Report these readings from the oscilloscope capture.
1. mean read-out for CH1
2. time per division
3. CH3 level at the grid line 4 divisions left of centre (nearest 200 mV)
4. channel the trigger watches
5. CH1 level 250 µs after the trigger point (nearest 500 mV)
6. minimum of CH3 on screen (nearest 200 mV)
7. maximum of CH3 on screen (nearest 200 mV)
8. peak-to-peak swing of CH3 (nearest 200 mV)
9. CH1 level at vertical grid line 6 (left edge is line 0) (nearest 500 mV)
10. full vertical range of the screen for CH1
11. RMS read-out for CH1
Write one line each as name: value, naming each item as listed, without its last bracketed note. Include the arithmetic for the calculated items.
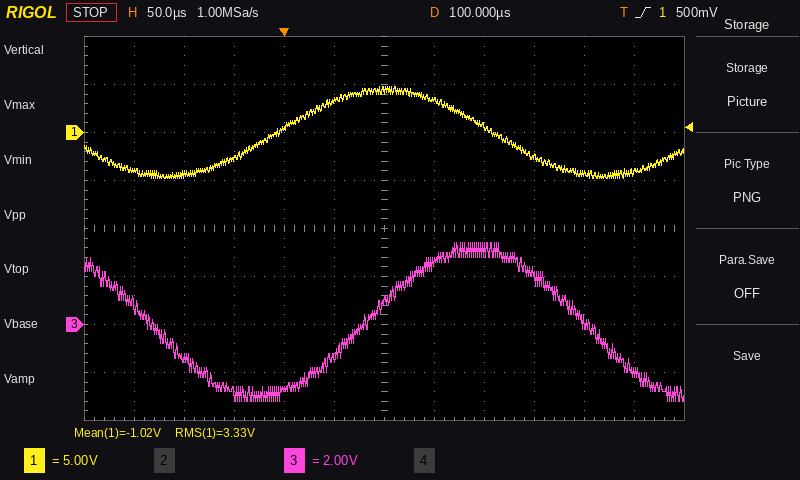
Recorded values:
mean read-out for CH1: -1.02 V
time per division: 50 µs
CH3 level at the grid line 4 divisions left of centre: -1.4 V
channel the trigger watches: CH1
CH1 level 250 µs after the trigger point: -2.5 V
minimum of CH3 on screen: -3.2 V
maximum of CH3 on screen: 3.4 V
peak-to-peak swing of CH3: 3.4 V − (-3.2 V) = 6.6 V
CH1 level at vertical grid line 6 (left edge is line 0): 4.5 V
full vertical range of the screen for CH1: 40 V
RMS read-out for CH1: 3.33 V
